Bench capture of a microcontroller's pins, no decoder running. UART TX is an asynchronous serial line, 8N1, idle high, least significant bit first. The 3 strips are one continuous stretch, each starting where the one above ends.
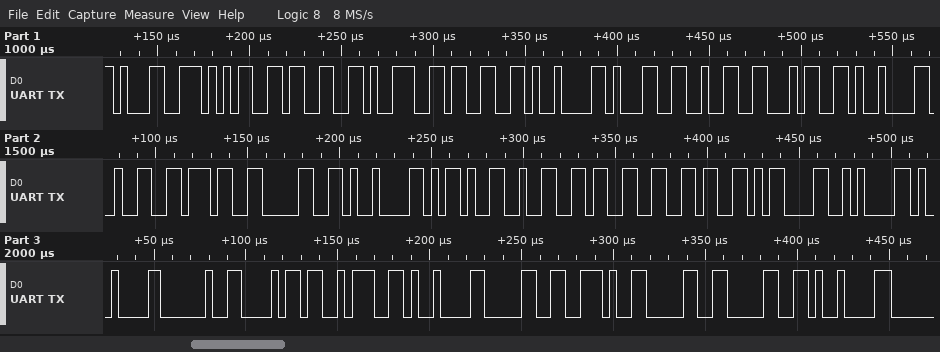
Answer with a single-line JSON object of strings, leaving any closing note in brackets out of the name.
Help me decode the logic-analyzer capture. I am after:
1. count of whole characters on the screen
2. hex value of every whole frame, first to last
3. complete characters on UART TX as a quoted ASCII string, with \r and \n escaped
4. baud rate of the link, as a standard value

{"count of whole characters on the screen": "30", "hex value of every whole frame, first to last": "31 35 33 39 33 09 31 32 34 09 32 37 30 09 2D 32 33 36 0D 0A 09 20 68 3A 09 30 2E 30 30 09", "complete characters on UART TX as a quoted ASCII string, with \\r and \\n escaped": "\"15393\\t124\\t270\\t-236\\r\\n\\t h:\\t0.00\\t\"", "baud rate of the link, as a standard value": "250000 baud"}
